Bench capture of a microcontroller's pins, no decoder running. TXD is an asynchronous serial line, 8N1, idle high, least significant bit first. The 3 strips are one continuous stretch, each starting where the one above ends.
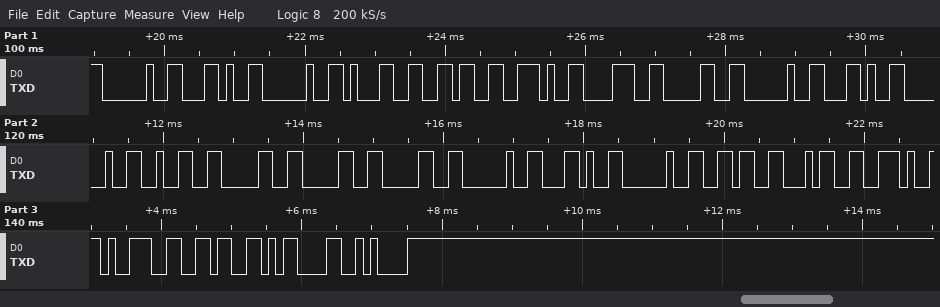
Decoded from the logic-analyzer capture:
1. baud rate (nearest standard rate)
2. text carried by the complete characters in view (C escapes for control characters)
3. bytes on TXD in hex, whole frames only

9600 baud
" , 16.80 , 2000 , 64.96\r\n"
0x20 0x2C 0x20 0x31 0x36 0x2E 0x38 0x30 0x20 0x2C 0x20 0x32 0x30 0x30 0x30 0x20 0x2C 0x20 0x36 0x34 0x2E 0x39 0x36 0x0D 0x0A
